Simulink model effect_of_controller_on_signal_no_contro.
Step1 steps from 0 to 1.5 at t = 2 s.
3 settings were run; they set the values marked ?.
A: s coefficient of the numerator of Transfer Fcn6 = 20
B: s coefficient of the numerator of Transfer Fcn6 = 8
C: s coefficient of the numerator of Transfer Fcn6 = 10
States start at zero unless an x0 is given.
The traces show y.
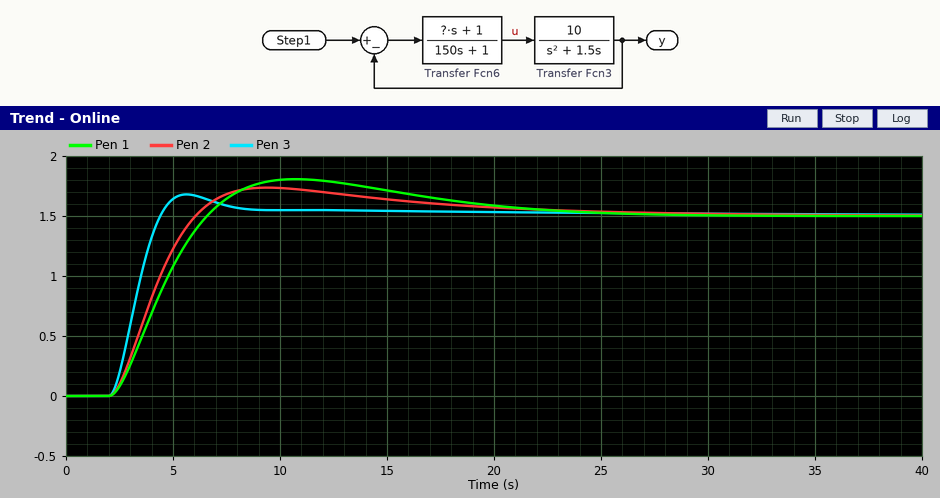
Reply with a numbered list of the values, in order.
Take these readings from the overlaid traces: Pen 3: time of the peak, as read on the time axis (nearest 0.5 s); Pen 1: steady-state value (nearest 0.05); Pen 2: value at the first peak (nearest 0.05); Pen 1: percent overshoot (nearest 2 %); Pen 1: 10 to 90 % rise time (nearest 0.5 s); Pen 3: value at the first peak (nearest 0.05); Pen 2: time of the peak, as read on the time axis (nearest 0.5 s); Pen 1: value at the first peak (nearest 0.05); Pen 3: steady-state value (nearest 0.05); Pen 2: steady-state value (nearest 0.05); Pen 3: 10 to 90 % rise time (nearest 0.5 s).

1. 5.5 s
2. 1.50
3. 1.75
4. 20 %
5. 3.0 s
6. 1.70
7. 9.5 s
8. 1.80
9. 1.50
10. 1.50
11. 1.5 s
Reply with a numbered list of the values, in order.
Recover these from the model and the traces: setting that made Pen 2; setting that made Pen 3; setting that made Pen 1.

1. C
2. A
3. B
